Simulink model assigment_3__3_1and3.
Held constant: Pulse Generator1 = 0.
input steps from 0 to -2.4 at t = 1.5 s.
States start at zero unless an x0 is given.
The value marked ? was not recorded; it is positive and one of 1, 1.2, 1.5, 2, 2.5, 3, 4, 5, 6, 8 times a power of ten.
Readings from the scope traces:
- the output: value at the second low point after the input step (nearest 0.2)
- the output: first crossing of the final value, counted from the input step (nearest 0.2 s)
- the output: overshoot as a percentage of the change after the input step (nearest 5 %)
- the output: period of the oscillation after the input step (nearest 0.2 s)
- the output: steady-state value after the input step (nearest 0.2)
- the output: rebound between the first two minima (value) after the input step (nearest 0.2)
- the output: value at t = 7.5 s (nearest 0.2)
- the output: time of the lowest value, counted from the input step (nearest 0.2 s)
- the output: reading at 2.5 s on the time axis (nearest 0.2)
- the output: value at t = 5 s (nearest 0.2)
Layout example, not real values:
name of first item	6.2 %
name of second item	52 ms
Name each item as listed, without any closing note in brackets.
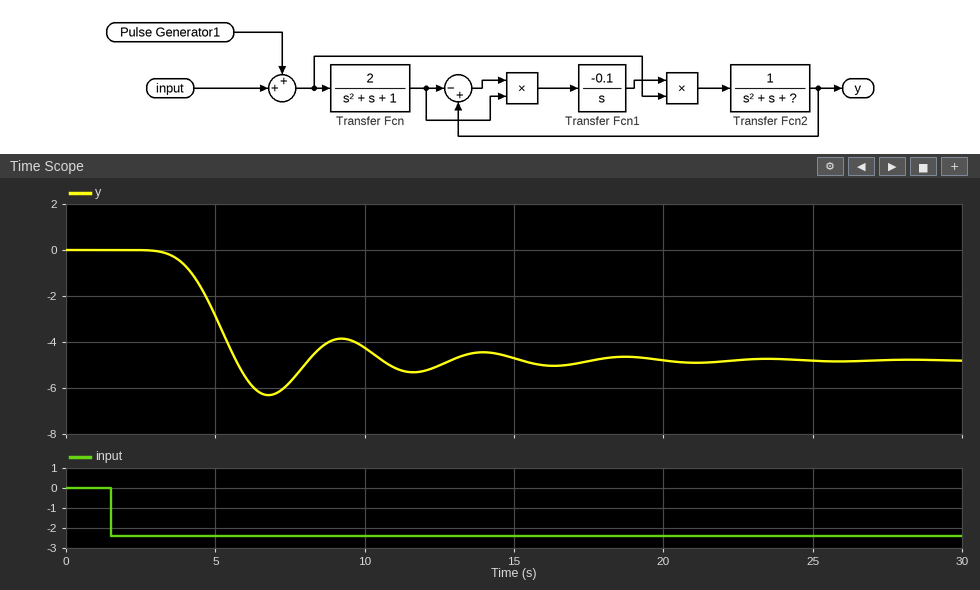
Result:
the output: value at the second low point after the input step	-5.4
the output: first crossing of the final value, counted from the input step	4.2 s
the output: overshoot as a percentage of the change after the input step	30 %
the output: period of the oscillation after the input step	4.8 s
the output: steady-state value after the input step	-4.8
the output: rebound between the first two minima (value) after the input step	-3.8
the output: value at t = 7.5 s	-5.8
the output: time of the lowest value, counted from the input step	5.2 s
the output: reading at 2.5 s on the time axis	0.0
the output: value at t = 5 s	-2.8
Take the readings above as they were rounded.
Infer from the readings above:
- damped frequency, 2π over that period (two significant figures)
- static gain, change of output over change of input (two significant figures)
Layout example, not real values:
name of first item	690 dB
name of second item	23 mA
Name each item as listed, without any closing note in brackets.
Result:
damped frequency, 2π over that period	1.3 rad/s
static gain, change of output over change of input	2.0
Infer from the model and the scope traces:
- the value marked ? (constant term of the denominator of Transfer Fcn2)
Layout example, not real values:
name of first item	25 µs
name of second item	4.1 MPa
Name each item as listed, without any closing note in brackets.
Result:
the value marked ?	2
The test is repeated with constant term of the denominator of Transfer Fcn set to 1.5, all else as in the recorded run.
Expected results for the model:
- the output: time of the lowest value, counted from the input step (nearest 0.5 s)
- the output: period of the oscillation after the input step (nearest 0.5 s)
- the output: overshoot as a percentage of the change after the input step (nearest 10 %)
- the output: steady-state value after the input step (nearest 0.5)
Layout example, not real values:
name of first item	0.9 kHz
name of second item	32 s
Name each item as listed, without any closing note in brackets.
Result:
the output: time of the lowest value, counted from the input step	5.0 s
the output: period of the oscillation after the input step	5.0 s
the output: overshoot as a percentage of the change after the input step	20 %
the output: steady-state value after the input step	-3.0
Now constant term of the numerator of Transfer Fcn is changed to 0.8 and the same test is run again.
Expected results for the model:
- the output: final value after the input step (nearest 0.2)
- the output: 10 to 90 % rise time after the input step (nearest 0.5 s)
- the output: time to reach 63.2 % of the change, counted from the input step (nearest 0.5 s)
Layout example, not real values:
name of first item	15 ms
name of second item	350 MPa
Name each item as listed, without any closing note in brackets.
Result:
the output: final value after the input step	-2.0
the output: 10 to 90 % rise time after the input step	7.5 s
the output: time to reach 63.2 % of the change, counted from the input step	5.0 s
